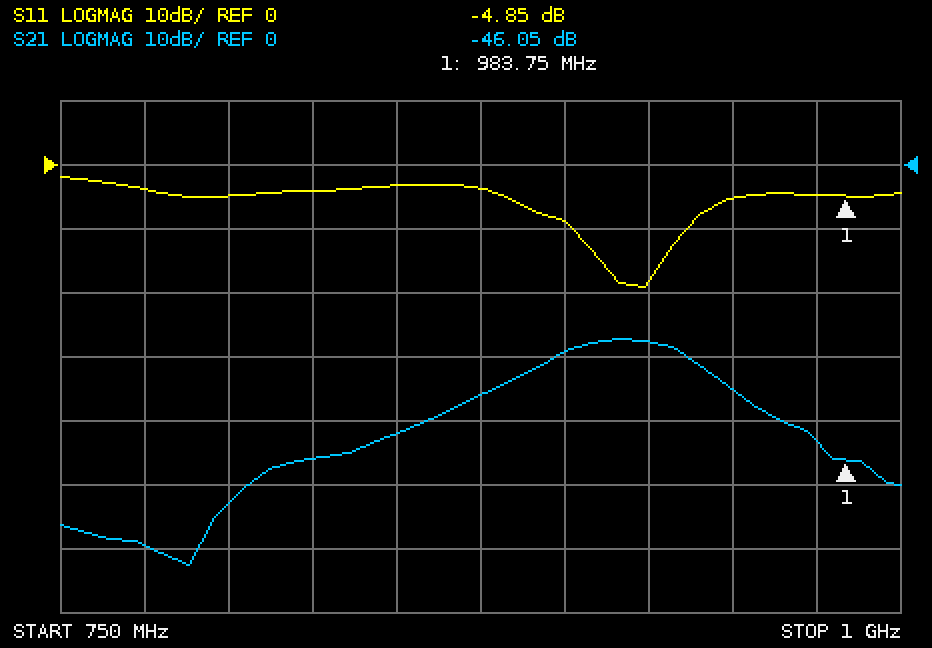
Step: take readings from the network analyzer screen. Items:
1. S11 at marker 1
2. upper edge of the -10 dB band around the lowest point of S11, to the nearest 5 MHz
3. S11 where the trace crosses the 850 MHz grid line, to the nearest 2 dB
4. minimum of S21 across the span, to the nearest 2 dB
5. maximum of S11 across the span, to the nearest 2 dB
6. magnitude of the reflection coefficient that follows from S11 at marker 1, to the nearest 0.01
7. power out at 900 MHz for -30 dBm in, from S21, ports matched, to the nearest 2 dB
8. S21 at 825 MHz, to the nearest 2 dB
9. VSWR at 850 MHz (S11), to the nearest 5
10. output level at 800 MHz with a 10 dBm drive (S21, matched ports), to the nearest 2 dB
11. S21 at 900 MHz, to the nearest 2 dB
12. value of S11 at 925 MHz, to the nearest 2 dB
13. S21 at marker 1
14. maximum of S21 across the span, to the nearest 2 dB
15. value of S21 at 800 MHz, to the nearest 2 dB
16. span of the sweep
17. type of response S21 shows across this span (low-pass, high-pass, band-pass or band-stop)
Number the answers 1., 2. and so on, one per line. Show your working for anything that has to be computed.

1. -4.85 dB
2. 935 MHz
3. -4 dB
4. -62 dB
5. -2 dB
6. 10^(-4.85/20) ≈ 0.57
7. -30 dBm + (-30 dB) = -60 dBm
8. -46 dB
9. |Γ| = 10^(-4/20) = 0.6310; VSWR = (1 + 0.6310)/(1 − 0.6310) ≈ 4.42, so 5 to the nearest 5
10. 10 dBm + (-52 dB) = -42 dBm
11. -30 dB
12. -18 dB
13. -46.05 dB
14. -28 dB
15. -52 dB
16. 250 MHz
17. band-pass
